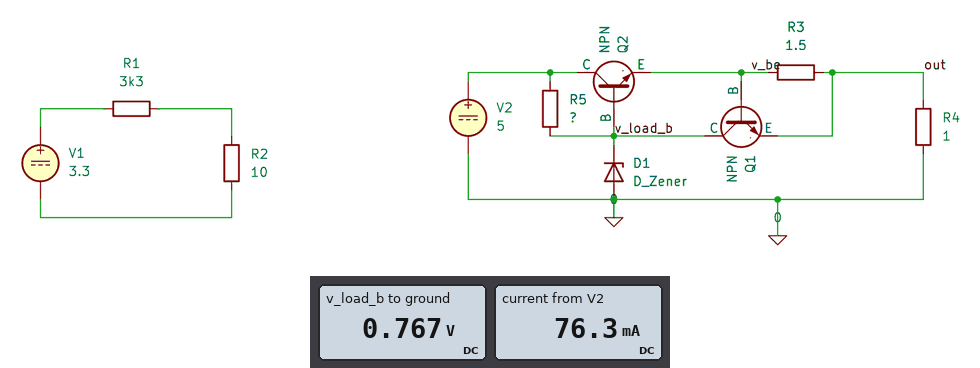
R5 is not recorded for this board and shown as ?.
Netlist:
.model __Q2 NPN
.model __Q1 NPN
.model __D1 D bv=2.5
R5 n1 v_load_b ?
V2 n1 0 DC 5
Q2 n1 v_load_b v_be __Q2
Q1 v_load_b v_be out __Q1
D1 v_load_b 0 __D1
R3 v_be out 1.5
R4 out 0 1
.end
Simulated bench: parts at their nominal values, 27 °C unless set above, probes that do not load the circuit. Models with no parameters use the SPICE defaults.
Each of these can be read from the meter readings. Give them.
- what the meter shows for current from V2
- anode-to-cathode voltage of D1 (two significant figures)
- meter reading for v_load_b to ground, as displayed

76.3 mA
770 mV
0.767 V
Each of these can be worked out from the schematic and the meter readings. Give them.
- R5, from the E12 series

56 Ω
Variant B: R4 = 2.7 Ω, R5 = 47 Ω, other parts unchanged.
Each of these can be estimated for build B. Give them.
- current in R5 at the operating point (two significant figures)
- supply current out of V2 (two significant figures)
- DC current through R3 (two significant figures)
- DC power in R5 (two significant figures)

90 mA
91 mA
800 µA
380 mW
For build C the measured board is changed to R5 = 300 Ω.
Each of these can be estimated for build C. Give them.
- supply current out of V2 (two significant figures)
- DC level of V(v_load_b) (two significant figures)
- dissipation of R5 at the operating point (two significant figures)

14 mA
720 mV
61 mW
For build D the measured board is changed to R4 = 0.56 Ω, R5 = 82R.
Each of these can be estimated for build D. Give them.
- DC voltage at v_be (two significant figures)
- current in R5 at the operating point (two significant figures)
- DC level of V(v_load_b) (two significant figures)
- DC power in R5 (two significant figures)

1.0 mV
52 mA
760 mV
220 mW
